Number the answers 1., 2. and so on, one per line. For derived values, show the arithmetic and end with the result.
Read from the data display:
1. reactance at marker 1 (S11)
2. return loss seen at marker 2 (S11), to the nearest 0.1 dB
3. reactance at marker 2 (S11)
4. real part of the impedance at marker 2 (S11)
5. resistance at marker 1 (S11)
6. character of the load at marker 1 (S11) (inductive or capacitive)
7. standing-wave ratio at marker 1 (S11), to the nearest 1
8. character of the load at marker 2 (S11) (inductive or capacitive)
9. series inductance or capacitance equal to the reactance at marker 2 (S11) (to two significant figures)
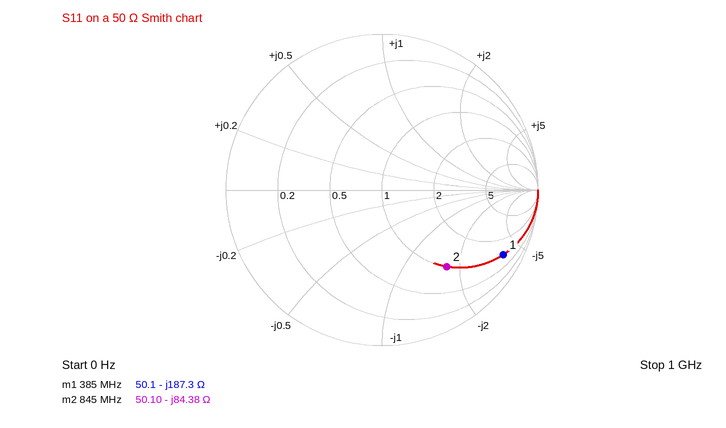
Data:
1. -187.3 Ω
2. 3.8 dB
3. -84.38 Ω
4. 50.10 Ω
5. 50.1 Ω
6. capacitive
7. 16
8. capacitive
9. C = 1/(2π × 845 MHz × 84.38 Ω) ≈ 2.2 pF
